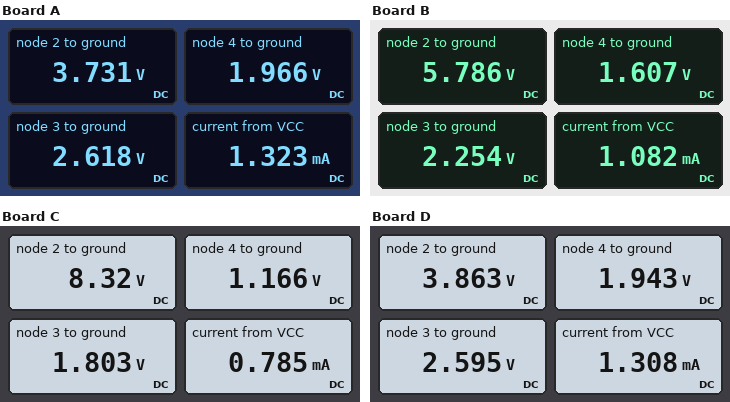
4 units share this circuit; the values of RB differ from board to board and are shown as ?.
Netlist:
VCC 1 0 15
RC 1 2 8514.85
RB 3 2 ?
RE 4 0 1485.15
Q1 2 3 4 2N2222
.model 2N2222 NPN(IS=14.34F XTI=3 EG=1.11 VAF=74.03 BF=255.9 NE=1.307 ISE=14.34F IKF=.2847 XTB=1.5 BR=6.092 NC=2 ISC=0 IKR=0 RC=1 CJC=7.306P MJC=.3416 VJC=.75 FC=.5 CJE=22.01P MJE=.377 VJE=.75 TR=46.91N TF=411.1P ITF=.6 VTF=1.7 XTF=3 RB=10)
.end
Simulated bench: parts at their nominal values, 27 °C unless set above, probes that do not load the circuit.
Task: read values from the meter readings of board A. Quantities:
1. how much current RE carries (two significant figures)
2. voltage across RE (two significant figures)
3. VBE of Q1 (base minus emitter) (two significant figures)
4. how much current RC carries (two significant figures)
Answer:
1.3 mA
2.0 V
650 mV
1.3 mA
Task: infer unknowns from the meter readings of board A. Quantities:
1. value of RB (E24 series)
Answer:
130 kΩ
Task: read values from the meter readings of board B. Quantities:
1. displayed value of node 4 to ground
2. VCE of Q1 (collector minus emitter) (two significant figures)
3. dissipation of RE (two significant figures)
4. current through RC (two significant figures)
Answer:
1.607 V
4.2 V
1.7 mW
1.1 mA
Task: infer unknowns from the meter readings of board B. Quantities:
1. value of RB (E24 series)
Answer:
510 kΩ
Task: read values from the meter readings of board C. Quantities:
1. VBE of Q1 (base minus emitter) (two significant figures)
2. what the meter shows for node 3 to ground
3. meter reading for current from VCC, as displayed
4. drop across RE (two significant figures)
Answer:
640 mV
1.803 V
0.785 mA
1.2 V
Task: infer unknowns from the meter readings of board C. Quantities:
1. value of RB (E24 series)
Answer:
1.3 MΩ
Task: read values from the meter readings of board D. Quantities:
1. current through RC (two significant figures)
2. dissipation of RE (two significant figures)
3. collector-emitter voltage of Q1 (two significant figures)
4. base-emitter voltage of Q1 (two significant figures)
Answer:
1.3 mA
2.5 mW
1.9 V
650 mV
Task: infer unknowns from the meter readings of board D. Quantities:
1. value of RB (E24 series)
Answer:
150 kΩ
